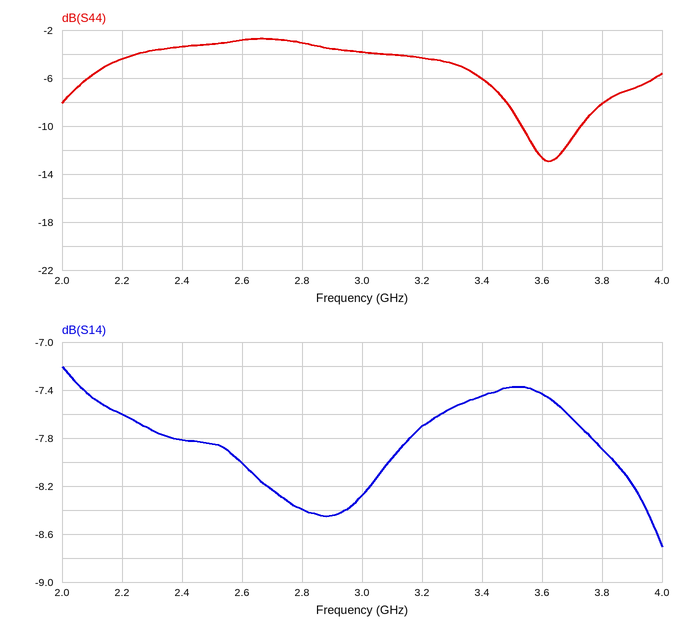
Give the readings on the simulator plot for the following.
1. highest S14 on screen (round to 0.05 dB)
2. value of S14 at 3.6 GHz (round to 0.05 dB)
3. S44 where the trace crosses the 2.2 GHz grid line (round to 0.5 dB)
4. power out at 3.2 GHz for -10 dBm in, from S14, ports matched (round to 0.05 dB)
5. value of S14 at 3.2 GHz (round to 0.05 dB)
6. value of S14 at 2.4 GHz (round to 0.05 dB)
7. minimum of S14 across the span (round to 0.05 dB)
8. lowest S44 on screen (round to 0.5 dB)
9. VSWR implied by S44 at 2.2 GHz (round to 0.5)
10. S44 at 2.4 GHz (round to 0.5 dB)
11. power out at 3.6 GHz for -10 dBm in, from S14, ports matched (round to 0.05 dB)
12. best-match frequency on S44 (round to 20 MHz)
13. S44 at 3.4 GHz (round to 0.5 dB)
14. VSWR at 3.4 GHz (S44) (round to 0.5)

-7.20 dB
-7.45 dB
-4.5 dB
-17.70 dBm
-7.70 dB
-7.80 dB
-8.70 dB
-13.0 dB
4.0
-3.5 dB
-17.45 dBm
3.62 GHz
-6.0 dB
3.0
